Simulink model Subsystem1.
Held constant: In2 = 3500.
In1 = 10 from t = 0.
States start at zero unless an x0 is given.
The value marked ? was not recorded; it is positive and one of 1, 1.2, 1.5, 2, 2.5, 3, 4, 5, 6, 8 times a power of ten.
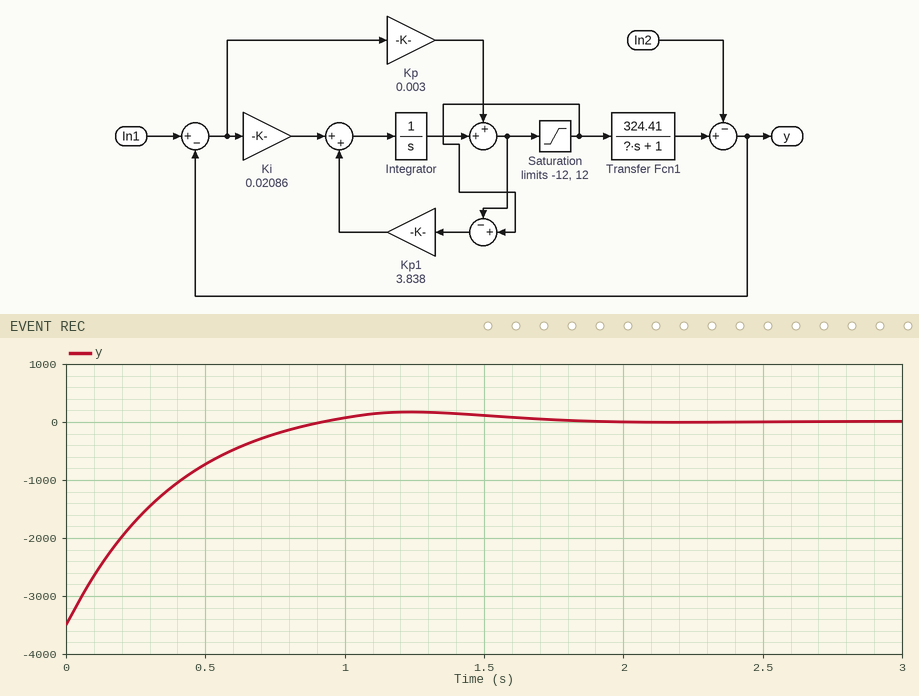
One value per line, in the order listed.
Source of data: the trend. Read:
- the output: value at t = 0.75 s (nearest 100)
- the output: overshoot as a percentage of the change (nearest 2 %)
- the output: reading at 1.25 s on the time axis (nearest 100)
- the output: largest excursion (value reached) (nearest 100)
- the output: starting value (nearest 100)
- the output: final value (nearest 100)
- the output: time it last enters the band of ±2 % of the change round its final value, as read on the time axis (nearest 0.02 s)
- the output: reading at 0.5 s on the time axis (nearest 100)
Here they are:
-200
4 %
200
200
-3500
0
1.60 s
-700
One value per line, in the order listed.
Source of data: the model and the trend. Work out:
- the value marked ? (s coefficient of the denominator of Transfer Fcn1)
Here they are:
0.4
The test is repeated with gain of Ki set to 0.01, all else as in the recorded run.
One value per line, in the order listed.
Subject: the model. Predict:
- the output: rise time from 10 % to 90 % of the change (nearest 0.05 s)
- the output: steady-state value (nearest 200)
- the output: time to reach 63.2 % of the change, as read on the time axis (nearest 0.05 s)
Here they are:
0.65 s
0
0.35 s
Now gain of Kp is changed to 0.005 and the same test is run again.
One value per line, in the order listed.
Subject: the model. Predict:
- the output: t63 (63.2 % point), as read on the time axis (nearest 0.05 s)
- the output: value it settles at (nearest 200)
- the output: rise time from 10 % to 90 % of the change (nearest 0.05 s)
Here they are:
0.35 s
0
0.65 s
